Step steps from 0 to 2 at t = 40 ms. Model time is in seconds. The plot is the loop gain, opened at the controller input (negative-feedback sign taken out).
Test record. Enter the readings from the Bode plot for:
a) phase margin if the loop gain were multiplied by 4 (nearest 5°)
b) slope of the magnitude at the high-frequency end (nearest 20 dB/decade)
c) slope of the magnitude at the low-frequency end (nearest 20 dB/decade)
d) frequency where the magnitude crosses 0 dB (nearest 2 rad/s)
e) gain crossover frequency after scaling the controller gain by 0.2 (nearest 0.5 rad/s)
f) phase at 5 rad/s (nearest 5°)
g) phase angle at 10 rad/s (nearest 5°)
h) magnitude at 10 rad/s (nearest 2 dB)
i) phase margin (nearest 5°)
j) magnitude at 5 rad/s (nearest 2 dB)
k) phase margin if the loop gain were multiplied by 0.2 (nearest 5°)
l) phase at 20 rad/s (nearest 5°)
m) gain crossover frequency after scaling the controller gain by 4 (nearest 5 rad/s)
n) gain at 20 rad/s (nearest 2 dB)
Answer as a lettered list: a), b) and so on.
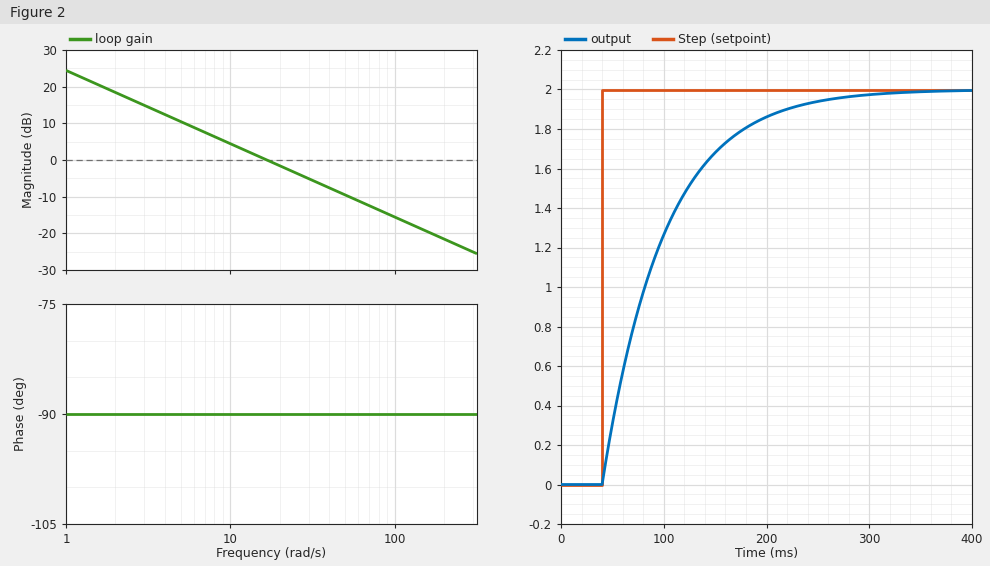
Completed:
a) 90°
b) -20 dB/decade
c) -20 dB/decade
d) 16 rad/s
e) 3.5 rad/s
f) -90°
g) -90°
h) 4 dB
i) 90°
j) 10 dB
k) 90°
l) -90°
m) 65 rad/s
n) -2 dB
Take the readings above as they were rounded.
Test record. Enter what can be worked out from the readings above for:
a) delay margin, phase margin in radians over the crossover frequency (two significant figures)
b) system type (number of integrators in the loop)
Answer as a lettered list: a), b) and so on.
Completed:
a) 0.098 s
b) 1
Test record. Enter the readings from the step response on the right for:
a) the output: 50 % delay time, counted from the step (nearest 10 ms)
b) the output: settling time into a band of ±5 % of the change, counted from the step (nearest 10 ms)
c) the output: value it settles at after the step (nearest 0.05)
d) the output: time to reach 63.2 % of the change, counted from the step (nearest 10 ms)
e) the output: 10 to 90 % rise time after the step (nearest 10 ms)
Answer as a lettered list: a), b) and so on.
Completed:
a) 40 ms
b) 180 ms
c) 2.00
d) 60 ms
e) 130 ms
